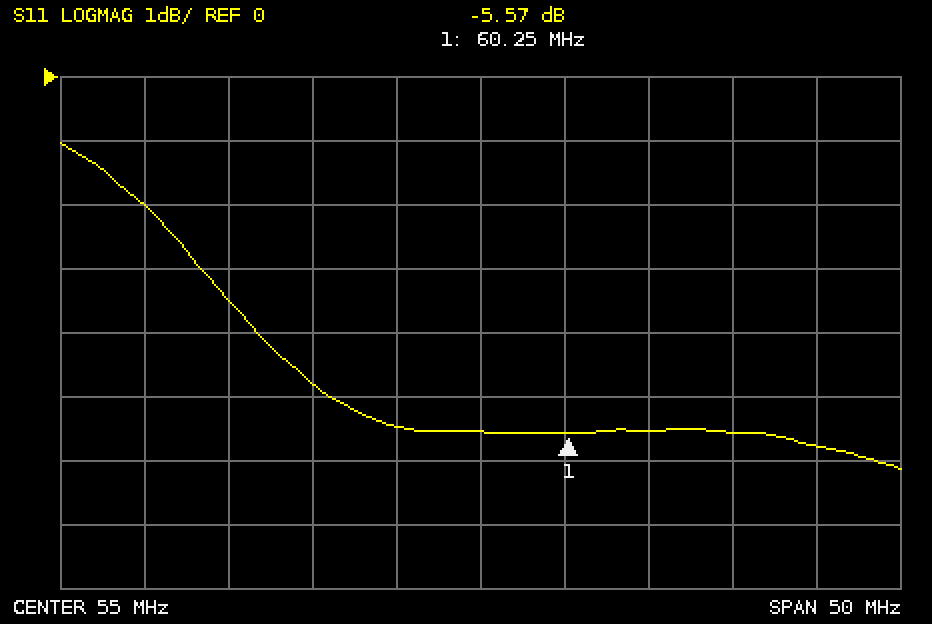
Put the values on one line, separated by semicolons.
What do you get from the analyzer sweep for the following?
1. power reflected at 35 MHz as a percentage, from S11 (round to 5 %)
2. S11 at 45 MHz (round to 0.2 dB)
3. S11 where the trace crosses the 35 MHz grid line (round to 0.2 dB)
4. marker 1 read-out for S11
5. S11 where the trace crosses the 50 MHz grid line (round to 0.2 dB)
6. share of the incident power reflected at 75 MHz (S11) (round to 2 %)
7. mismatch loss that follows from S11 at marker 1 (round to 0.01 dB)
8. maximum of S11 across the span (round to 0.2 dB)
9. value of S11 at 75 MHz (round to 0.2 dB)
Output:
65 %; -4.8 dB; -2.0 dB; -5.57 dB; -5.4 dB; 26 %; 1.41 dB; -1.0 dB; -5.8 dB
